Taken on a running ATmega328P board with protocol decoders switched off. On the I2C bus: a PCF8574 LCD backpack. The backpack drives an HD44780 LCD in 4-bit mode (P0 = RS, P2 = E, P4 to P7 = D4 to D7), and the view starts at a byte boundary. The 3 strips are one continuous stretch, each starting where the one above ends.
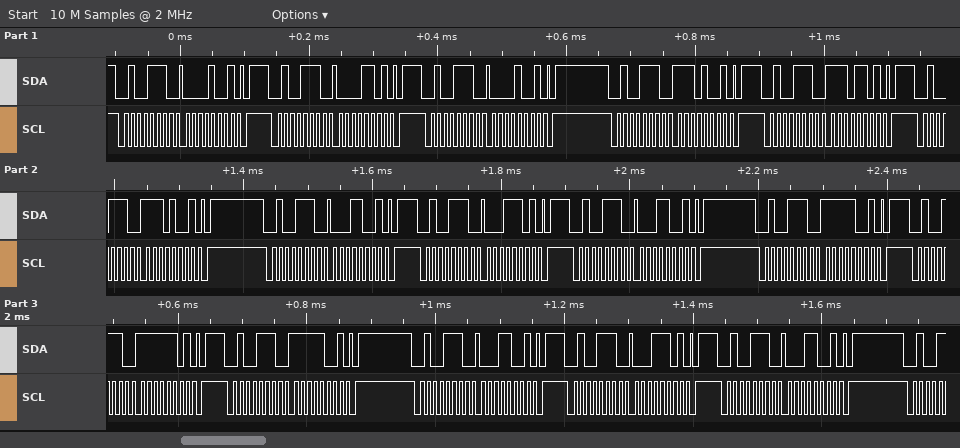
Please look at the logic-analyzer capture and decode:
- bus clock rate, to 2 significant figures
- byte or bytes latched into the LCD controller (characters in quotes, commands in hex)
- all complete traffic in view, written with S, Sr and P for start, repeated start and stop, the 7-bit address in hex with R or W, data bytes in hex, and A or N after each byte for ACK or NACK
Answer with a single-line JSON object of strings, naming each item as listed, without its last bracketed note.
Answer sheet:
{"bus clock rate, to 2 significant figures": "100 kHz", "byte or bytes latched into the LCD controller": "data 0x0E data 0x1F", "all complete traffic in view, written with S, Sr and P for start, repeated start and stop, the 7-bit address in hex with R or W, data bytes in hex, and A or N after each byte for ACK or NACK": "S 27W A 09 A P S 27W A 0D A P S 27W A 09 A P S 27W A E9 A P S 27W A ED A P S 27W A E9 A P S 27W A 19 A P S 27W A 1D A P S 27W A 19 A P S 27W A F9 A P S 27W A FD A P S 27W A F9 A P S 27W A 19 A P S 27W A 1D A P S 27W A 19 A P"}
